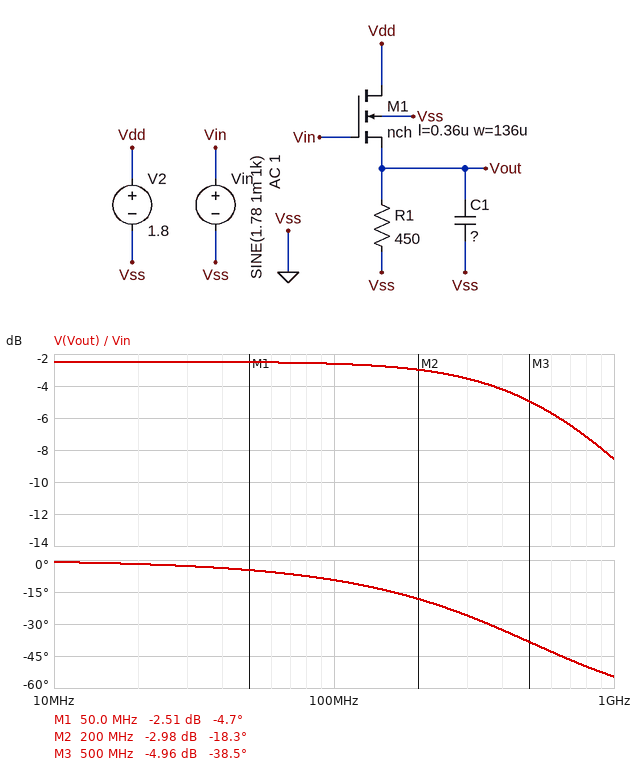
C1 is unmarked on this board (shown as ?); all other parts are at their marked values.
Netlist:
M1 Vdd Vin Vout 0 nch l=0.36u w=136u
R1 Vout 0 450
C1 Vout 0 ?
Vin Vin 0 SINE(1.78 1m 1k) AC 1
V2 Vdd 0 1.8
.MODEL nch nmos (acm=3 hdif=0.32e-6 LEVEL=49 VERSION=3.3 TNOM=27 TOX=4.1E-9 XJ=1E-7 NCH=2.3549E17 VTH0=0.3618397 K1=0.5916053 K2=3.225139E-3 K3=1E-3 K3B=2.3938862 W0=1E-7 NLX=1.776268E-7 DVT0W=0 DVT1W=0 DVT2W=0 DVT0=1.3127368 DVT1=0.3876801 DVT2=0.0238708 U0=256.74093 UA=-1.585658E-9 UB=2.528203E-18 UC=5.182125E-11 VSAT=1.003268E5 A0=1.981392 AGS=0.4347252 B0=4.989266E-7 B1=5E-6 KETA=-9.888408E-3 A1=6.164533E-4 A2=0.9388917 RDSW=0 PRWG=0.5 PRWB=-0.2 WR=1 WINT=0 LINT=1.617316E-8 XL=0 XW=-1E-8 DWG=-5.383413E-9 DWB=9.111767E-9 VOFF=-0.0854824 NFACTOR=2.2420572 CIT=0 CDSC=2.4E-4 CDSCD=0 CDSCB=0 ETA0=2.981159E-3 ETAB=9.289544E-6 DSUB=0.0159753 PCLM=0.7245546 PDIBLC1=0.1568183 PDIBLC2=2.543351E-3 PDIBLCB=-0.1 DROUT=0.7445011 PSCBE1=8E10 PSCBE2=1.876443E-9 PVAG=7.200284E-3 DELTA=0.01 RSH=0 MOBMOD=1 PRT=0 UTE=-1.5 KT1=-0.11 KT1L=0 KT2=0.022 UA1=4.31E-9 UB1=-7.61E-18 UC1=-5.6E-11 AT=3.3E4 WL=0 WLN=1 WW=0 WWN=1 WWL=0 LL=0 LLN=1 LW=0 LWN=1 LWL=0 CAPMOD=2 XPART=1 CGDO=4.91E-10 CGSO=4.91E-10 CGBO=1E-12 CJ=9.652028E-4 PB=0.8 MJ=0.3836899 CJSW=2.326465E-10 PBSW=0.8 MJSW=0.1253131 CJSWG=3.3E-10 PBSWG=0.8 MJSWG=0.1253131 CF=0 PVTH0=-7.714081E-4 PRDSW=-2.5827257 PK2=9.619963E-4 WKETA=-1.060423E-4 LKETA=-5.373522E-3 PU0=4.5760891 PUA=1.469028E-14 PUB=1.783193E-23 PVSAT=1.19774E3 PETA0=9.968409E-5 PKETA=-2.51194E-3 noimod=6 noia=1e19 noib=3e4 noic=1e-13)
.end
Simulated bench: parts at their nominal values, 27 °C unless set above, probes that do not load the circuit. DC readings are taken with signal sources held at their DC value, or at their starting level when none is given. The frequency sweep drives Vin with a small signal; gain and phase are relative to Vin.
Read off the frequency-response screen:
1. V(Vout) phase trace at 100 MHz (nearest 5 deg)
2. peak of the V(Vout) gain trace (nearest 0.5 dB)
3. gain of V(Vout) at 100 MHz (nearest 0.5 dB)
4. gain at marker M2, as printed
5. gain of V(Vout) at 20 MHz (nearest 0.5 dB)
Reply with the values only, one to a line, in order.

-10 deg
-2.5 dB
-2.5 dB
-2.98 dB
-2.5 dB
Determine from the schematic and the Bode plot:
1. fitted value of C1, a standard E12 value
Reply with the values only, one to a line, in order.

6.8 pF
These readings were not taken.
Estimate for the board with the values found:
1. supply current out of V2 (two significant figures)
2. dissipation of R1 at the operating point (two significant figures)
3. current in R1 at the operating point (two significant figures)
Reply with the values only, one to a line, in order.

2.0 mA
1.8 mW
2.0 mA
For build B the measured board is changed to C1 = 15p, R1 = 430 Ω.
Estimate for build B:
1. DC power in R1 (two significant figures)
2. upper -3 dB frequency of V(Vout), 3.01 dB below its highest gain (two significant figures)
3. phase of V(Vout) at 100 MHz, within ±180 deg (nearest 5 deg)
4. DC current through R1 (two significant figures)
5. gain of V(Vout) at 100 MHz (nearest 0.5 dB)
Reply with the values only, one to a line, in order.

1.9 mW
270 MHz
-20 deg
2.1 mA
-3.0 dB
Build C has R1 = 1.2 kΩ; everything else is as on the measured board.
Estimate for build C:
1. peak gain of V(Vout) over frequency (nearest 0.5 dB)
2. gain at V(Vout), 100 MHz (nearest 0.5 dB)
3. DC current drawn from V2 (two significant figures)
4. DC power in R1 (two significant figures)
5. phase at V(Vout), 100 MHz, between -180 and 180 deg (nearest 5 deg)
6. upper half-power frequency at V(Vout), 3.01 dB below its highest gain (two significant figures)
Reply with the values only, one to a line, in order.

-2.0 dB
-2.5 dB
810 µA
780 µW
-15 deg
340 MHz
